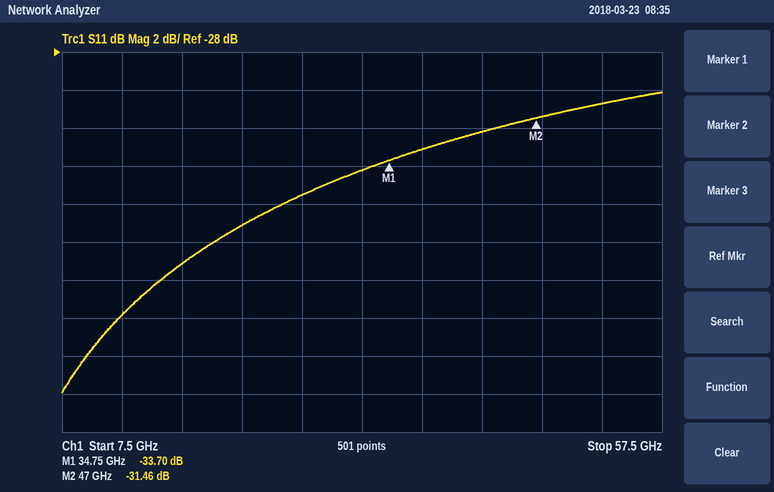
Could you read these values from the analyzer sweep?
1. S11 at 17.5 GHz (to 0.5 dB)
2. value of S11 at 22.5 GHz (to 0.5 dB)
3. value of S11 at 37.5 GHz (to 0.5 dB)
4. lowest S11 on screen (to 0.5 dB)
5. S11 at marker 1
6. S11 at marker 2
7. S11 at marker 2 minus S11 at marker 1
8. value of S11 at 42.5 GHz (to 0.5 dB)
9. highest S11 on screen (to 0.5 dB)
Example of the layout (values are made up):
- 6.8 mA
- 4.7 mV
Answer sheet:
- -39.0 dB
- -37.0 dB
- -33.0 dB
- -46.0 dB
- -33.70 dB
- -31.46 dB
- 2.24 dB
- -32.0 dB
- -30.0 dB
